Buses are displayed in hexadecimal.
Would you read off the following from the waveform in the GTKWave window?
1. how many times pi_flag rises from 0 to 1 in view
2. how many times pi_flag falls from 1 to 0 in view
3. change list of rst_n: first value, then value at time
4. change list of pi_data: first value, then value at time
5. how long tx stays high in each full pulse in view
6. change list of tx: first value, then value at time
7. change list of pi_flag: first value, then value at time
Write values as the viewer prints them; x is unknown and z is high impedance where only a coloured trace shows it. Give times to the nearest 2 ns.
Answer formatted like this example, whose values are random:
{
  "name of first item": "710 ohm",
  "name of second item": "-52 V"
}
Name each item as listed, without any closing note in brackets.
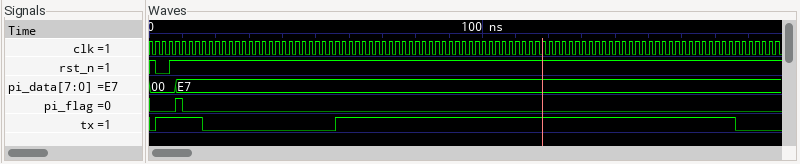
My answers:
{
  "how many times pi_flag rises from 0 to 1 in view": "1",
  "how many times pi_flag falls from 1 to 0 in view": "1",
  "change list of rst_n: first value, then value at time": "1, 0 at 2 ns, 1 at 6 ns",
  "change list of pi_data: first value, then value at time": "00, E7 at 8 ns",
  "how long tx stays high in each full pulse in view": "14 ns, 120 ns",
  "change list of tx: first value, then value at time": "0, 1 at 2 ns, 0 at 16 ns, 1 at 56 ns, 0 at 176 ns",
  "change list of pi_flag: first value, then value at time": "0, 1 at 8 ns, 0 at 10 ns"
}
